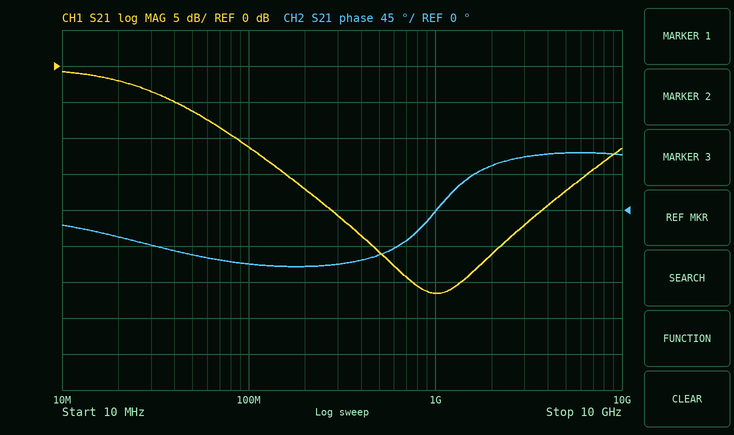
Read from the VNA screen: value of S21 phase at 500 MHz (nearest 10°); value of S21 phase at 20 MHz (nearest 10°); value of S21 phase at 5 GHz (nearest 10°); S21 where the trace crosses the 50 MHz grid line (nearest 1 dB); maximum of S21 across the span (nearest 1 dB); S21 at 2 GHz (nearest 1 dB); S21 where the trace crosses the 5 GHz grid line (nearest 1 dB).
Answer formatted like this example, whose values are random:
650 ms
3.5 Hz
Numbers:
-60°
-30°
70°
-6 dB
-1 dB
-26 dB
-17 dB
